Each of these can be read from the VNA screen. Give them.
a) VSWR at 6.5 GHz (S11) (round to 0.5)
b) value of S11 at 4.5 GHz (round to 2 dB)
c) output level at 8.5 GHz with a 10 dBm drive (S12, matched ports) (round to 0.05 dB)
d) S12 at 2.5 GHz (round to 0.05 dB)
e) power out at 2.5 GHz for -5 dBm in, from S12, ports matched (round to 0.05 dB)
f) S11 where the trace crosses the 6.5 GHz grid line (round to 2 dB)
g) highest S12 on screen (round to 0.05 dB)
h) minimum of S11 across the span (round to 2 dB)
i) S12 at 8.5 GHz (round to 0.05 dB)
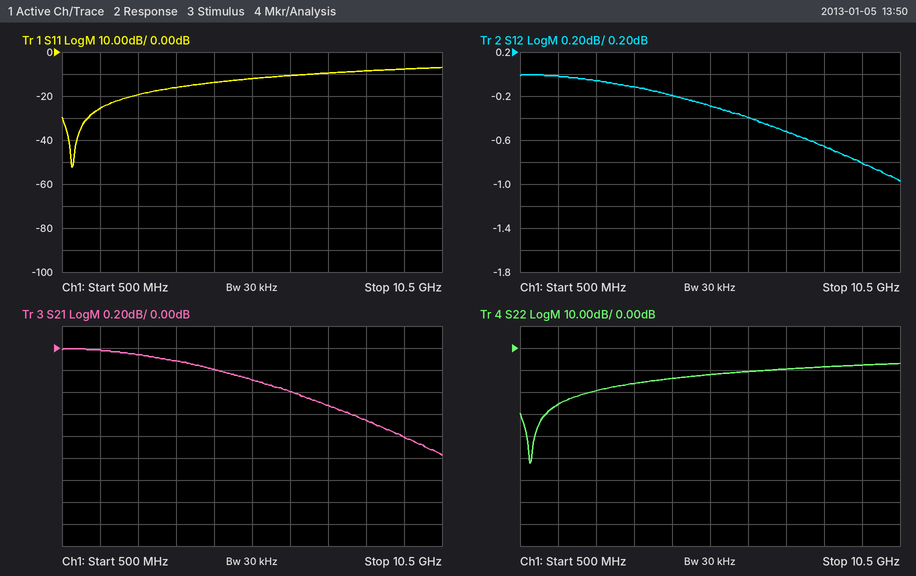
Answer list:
2.0
-14 dB
9.35 dBm
-0.05 dB
-5.05 dBm
-10 dB
0.00 dB
-52 dB
-0.65 dB
